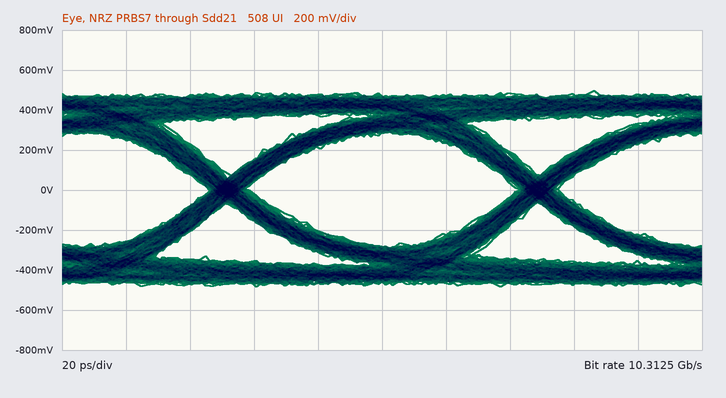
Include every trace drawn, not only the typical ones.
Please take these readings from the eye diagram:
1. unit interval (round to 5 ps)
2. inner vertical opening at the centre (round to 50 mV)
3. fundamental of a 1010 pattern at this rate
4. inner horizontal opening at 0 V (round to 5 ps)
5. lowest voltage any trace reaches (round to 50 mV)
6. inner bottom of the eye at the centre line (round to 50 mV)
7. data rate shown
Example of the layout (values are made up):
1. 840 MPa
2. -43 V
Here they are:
1. 95 ps
2. 550 mV
3. 5.15625 GHz
4. 85 ps
5. -500 mV
6. -300 mV
7. 10.3125 Gb/s
